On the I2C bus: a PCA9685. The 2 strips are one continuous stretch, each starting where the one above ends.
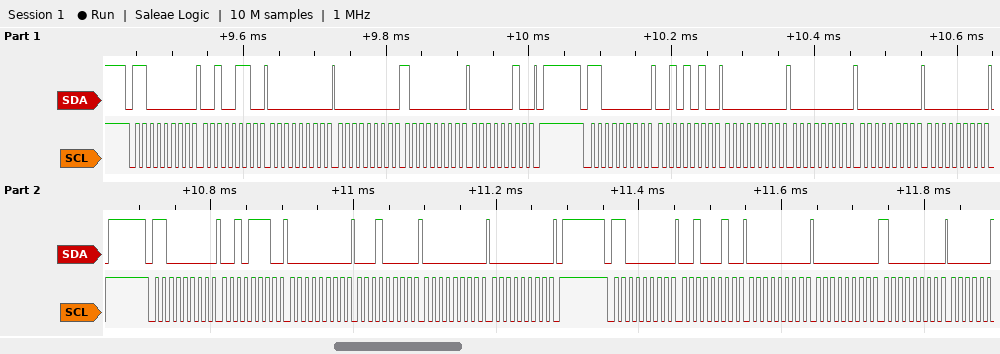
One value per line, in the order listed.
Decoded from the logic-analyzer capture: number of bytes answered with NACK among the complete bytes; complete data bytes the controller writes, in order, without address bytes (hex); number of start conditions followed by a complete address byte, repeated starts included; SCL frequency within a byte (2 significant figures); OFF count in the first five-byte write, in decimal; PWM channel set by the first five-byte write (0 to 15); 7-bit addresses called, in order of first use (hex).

0
26 00 00 80 02 2A 00 00 00 00 2E 00 10 00 00 22 00 00 80
4
100 kHz
640
8
0x60
